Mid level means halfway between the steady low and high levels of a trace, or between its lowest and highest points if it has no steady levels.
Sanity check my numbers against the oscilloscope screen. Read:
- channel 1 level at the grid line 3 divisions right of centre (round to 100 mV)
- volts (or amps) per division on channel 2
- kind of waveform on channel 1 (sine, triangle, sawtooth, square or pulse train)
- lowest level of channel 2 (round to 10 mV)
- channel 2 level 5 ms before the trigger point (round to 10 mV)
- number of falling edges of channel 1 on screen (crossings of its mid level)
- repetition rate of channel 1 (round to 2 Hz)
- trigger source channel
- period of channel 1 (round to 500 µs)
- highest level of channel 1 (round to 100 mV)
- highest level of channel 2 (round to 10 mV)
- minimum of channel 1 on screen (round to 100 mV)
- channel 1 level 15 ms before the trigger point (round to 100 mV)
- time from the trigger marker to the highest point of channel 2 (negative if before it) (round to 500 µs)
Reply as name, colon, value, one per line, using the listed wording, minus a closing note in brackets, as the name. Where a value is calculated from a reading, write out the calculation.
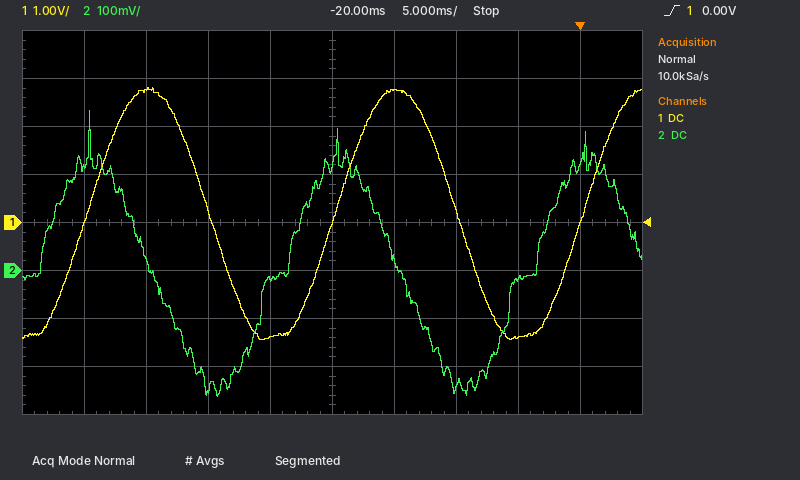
channel 1 level at the grid line 3 divisions right of centre: -2.4 V
volts (or amps) per division on channel 2: 100 mV
kind of waveform on channel 1: sine
lowest level of channel 2: -260 mV
channel 2 level 5 ms before the trigger point: -20 mV
number of falling edges of channel 1 on screen: 2
repetition rate of channel 1: 1 / 20.0 ms ≈ 50 Hz
trigger source channel: channel 1
period of channel 1: 20.0 ms
highest level of channel 1: 2.8 V
highest level of channel 2: 330 mV
minimum of channel 1 on screen: -2.4 V
channel 1 level 15 ms before the trigger point: 2.8 V
time from the trigger marker to the highest point of channel 2 (negative if before it): -39.5 ms
